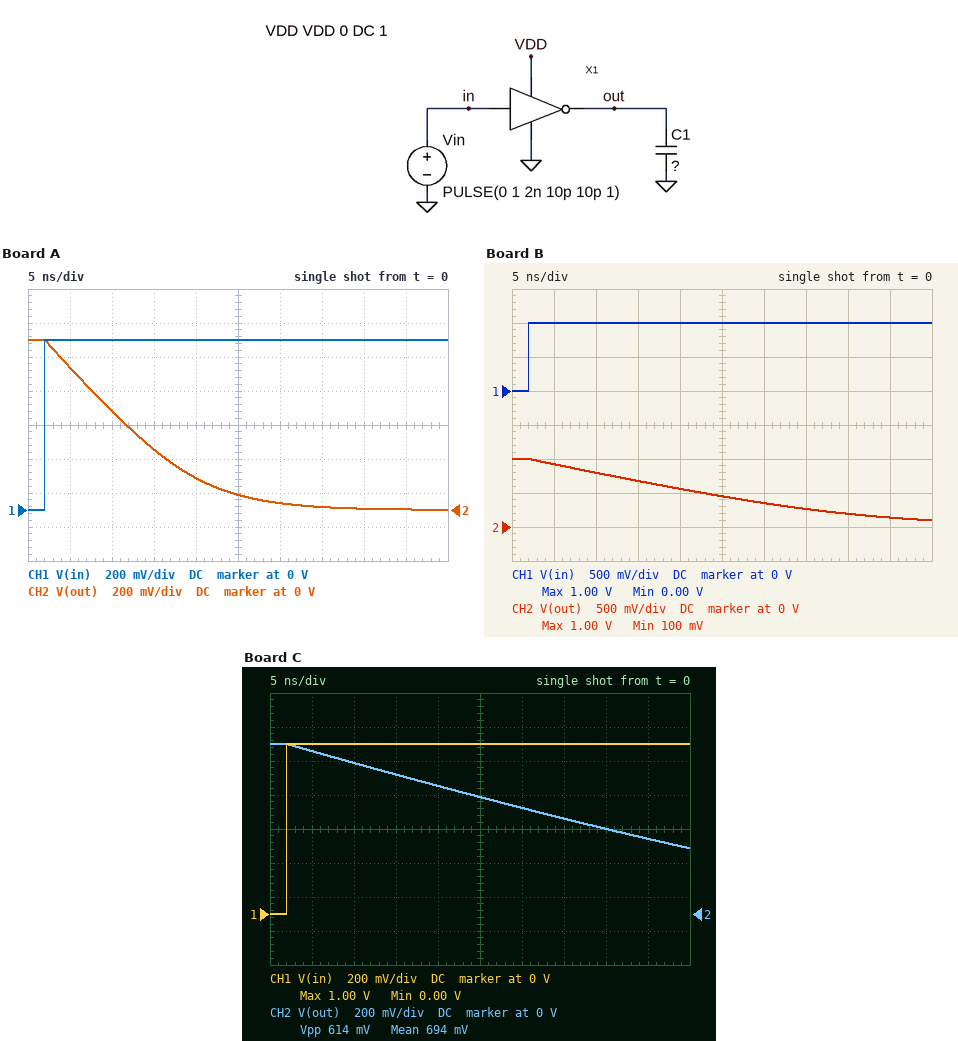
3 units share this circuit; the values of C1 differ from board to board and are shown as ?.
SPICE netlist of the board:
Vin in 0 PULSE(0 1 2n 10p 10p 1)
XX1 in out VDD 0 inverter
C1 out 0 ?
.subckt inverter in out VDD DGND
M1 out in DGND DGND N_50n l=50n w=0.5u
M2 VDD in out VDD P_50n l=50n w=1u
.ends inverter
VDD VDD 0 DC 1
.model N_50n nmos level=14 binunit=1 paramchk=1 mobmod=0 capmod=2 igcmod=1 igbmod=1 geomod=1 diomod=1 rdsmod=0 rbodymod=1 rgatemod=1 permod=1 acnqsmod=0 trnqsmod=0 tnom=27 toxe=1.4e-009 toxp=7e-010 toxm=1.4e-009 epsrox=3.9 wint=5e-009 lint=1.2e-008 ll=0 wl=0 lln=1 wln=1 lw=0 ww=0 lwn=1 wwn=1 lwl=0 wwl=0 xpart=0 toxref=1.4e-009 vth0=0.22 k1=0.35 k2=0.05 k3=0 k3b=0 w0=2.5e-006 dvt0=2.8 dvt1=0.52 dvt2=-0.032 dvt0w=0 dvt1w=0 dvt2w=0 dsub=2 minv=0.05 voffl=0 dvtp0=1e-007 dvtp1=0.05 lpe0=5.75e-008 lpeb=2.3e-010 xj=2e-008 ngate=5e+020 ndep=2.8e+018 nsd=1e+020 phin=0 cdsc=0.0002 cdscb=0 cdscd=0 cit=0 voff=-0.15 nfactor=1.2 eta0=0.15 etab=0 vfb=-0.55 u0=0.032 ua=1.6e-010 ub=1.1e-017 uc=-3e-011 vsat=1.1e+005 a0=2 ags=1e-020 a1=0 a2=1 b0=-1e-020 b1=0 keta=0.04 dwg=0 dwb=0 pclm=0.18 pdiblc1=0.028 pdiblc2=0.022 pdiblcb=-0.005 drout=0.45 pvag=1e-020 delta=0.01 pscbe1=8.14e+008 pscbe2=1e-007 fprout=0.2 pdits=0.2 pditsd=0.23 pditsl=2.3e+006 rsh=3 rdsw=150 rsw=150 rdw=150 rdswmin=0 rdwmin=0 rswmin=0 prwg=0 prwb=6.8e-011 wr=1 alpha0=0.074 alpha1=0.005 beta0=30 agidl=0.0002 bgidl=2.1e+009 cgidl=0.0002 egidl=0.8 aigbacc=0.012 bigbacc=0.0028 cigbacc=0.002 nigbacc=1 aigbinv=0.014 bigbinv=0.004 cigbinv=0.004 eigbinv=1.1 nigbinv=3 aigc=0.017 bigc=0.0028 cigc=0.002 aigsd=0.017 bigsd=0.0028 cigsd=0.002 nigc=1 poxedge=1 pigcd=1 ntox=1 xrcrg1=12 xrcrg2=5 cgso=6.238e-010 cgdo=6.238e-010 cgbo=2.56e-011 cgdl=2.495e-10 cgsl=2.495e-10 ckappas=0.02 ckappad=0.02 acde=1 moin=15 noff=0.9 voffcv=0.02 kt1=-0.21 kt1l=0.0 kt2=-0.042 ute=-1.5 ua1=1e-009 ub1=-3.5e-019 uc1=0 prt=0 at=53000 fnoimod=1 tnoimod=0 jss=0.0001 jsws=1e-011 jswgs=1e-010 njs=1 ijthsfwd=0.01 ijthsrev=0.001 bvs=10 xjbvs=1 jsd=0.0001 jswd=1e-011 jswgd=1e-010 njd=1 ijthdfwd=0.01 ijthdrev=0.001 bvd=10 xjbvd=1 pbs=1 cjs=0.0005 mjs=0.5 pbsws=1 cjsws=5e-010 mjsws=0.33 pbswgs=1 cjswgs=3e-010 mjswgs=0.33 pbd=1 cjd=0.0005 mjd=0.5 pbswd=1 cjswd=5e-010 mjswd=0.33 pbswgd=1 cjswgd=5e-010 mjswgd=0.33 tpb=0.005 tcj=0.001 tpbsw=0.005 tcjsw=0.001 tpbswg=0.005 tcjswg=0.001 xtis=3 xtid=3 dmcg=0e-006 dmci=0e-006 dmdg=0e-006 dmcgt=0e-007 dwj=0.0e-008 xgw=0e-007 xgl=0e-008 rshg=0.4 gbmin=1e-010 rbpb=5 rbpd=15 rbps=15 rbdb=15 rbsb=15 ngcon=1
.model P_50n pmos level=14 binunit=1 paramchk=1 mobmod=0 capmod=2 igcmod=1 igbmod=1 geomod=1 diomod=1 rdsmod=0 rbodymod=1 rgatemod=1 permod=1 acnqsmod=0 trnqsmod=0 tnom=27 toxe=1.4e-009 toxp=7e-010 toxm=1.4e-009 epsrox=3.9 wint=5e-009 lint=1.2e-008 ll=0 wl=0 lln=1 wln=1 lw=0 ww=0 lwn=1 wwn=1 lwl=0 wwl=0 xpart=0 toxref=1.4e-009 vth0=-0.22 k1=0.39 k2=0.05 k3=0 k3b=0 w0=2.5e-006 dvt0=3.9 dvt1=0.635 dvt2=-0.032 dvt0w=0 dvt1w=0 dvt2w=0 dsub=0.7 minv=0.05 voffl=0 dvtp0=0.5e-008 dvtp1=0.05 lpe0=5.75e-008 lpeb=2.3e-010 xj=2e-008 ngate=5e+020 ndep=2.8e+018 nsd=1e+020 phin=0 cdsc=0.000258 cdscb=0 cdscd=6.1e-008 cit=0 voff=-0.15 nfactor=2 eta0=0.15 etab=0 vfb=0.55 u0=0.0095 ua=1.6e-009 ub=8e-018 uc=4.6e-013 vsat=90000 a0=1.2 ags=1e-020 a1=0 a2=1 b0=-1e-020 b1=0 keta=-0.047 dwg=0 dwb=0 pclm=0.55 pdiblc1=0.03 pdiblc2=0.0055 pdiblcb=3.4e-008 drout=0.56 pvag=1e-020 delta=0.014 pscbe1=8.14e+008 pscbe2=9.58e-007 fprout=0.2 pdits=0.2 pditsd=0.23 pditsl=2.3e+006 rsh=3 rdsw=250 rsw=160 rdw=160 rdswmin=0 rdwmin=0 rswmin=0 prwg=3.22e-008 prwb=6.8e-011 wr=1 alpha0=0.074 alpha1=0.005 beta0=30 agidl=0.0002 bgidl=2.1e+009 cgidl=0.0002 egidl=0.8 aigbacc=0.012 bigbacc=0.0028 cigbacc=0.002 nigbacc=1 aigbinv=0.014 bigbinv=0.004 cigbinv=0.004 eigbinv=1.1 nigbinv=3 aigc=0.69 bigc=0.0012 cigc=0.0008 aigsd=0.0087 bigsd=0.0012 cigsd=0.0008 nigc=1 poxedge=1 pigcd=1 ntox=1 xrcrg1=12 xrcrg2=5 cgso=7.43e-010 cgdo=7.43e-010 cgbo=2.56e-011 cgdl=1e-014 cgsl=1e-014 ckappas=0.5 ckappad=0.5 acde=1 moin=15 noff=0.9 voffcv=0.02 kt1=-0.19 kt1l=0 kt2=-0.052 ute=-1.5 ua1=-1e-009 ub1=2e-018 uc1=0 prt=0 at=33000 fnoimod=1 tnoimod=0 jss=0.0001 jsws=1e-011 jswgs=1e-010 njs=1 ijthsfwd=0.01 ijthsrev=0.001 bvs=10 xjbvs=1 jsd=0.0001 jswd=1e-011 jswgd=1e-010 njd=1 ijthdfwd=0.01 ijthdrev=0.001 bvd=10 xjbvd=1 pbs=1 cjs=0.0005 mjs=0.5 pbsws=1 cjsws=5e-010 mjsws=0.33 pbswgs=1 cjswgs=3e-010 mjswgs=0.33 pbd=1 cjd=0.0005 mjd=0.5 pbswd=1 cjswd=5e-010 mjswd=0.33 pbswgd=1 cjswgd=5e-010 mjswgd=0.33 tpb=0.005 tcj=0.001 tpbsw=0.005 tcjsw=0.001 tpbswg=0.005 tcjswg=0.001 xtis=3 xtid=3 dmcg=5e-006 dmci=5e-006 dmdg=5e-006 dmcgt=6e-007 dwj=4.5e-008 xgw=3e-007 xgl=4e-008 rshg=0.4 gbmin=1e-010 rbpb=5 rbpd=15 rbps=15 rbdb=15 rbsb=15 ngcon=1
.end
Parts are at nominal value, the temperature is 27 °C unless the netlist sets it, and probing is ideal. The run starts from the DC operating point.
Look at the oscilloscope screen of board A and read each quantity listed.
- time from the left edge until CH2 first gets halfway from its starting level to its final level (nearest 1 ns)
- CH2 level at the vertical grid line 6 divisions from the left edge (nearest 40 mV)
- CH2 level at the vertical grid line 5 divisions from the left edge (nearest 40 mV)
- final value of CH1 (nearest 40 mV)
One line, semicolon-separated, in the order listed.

12 ns; 40 mV; 80 mV; 1.00 V
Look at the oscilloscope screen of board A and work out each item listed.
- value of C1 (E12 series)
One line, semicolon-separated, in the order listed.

5.6 pF
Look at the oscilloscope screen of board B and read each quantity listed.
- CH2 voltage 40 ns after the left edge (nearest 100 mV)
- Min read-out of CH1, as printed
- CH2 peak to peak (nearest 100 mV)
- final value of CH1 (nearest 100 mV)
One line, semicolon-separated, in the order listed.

200 mV; 0.00 V; 900 mV; 1.0 V
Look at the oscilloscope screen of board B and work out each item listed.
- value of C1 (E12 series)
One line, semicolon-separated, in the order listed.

12 pF
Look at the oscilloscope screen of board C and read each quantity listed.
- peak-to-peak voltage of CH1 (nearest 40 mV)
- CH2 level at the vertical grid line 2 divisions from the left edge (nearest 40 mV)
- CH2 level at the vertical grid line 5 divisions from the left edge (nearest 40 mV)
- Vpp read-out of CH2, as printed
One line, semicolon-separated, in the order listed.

1.00 V; 880 mV; 680 mV; 614 mV
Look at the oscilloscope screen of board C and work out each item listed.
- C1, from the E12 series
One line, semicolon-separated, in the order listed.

22 pF
